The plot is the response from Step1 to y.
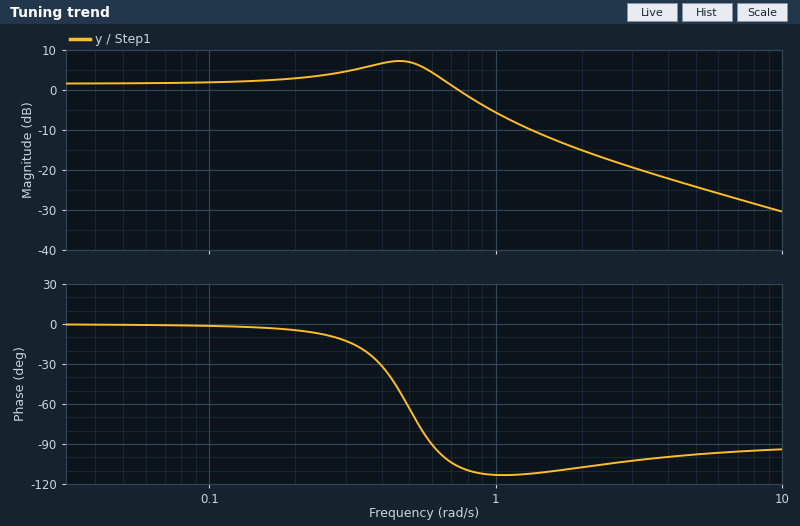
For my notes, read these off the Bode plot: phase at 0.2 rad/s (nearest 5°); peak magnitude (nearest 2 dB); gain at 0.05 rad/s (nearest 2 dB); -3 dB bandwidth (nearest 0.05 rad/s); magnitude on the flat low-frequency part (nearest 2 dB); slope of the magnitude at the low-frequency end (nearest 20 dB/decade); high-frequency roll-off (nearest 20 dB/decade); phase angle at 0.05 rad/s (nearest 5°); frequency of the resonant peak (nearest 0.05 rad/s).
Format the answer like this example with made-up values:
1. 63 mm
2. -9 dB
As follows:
1. -5°
2. 8 dB
3. 2 dB
4. 0.80 rad/s
5. 2 dB
6. 0 dB/decade
7. -20 dB/decade
8. 0°
9. 0.45 rad/s
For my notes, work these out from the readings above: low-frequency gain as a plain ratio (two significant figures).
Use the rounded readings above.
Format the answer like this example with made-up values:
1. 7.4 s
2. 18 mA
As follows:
1. 1.3
